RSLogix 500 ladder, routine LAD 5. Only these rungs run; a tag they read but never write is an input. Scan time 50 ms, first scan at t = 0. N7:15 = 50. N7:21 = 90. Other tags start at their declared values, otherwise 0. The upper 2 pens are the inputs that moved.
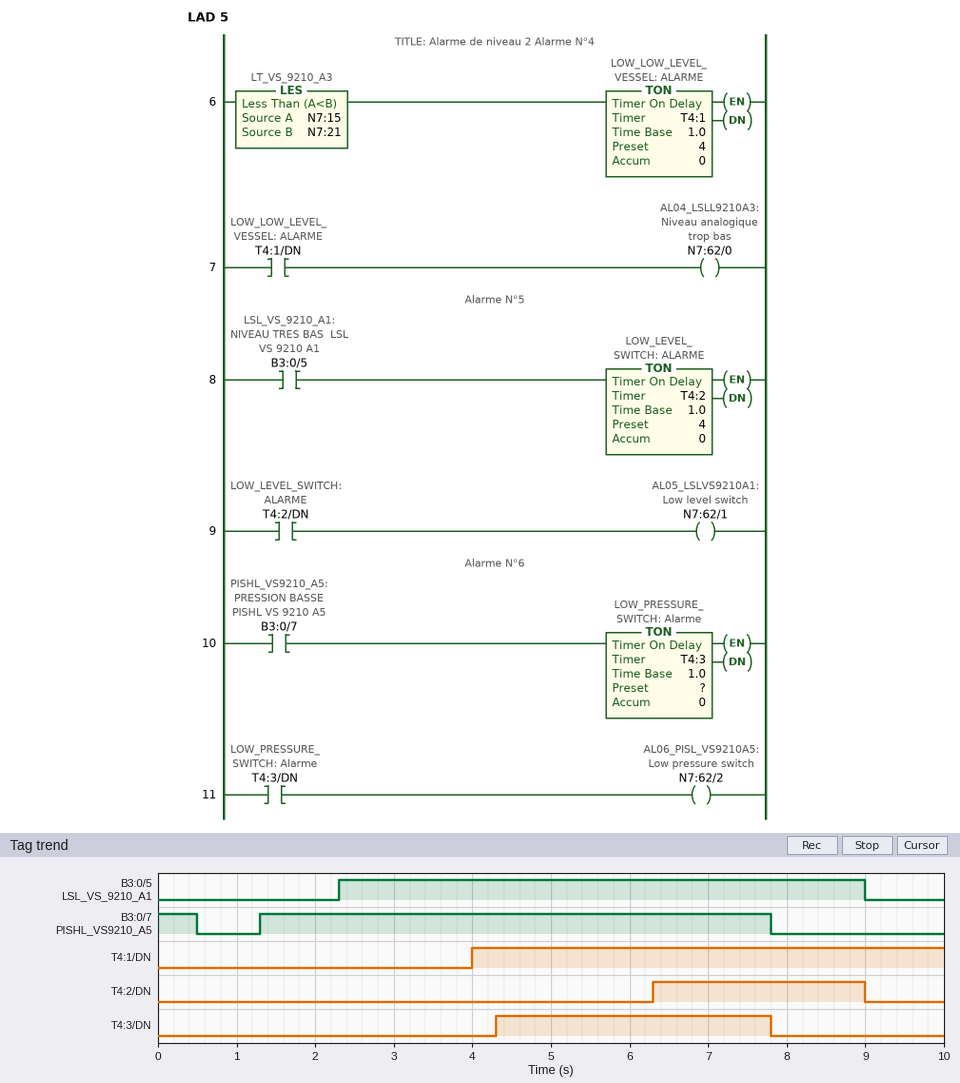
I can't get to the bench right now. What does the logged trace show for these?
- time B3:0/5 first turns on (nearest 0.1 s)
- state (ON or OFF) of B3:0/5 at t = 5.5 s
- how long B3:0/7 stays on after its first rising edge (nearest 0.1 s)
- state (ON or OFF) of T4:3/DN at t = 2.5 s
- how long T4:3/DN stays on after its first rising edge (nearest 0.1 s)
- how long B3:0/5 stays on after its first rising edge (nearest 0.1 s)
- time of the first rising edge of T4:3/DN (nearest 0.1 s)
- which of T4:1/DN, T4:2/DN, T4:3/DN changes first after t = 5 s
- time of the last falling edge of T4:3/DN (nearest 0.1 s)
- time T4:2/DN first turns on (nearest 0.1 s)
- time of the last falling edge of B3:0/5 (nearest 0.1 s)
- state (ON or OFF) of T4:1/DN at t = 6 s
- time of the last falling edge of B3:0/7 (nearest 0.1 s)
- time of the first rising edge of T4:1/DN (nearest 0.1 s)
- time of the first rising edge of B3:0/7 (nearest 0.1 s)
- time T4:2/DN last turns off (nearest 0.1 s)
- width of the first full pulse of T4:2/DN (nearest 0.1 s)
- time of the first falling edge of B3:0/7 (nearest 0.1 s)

2.3 s
ON
6.5 s
OFF
3.5 s
6.7 s
4.3 s
T4:2/DN
7.8 s
6.3 s
9.0 s
ON
7.8 s
4.0 s
1.3 s
9.0 s
2.7 s
0.5 s
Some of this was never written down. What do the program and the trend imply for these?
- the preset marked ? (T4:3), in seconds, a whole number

3 s
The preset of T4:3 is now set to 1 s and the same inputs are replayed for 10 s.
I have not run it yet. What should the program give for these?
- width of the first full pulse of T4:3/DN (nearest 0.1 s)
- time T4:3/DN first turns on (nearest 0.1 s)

5.5 s
2.3 s
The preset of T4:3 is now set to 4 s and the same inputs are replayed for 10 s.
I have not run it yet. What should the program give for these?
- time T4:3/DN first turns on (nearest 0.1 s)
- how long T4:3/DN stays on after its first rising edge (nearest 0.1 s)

5.3 s
2.5 s
